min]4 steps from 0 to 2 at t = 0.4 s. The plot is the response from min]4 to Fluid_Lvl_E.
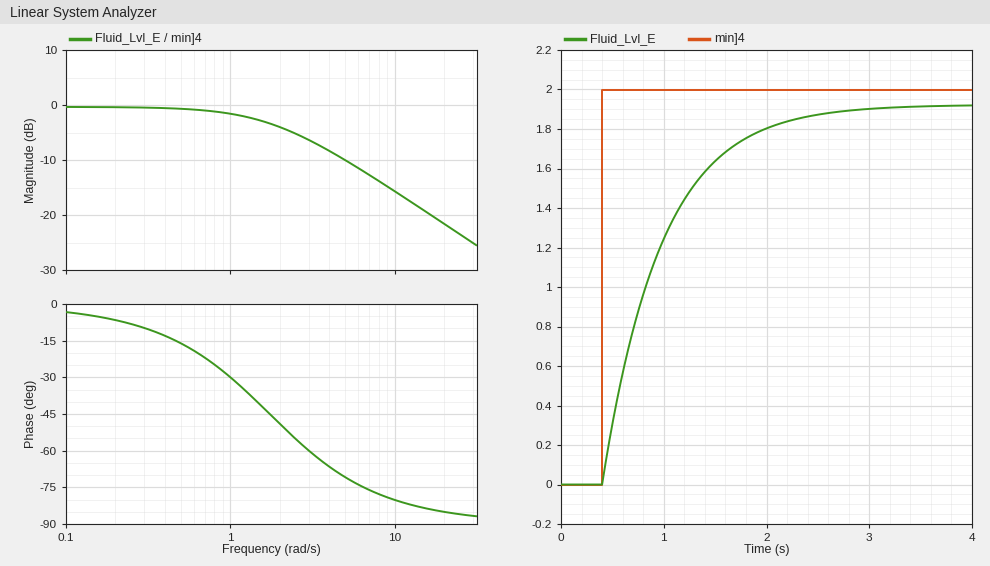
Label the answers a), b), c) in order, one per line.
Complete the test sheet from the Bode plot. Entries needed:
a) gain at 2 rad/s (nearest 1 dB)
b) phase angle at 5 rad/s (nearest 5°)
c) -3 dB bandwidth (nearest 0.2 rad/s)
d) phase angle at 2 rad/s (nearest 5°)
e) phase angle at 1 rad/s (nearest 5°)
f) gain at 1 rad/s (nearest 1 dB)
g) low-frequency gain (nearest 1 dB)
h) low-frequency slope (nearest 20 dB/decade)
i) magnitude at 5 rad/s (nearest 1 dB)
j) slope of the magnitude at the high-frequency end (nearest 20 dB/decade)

a) -4 dB
b) -70°
c) 1.8 rad/s
d) -50°
e) -30°
f) -2 dB
g) 0 dB
h) 0 dB/decade
i) -10 dB
j) -20 dB/decade
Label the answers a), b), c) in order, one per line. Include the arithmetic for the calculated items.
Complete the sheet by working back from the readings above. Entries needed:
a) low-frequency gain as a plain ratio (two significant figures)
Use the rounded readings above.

a) 10^(0 / 20) = 1.0
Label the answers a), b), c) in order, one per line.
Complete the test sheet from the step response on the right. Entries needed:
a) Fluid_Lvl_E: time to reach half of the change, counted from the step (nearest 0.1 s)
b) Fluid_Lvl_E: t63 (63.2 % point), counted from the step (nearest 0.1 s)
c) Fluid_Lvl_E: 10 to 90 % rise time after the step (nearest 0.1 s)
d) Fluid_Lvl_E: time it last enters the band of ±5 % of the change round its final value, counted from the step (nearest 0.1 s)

a) 0.4 s
b) 0.6 s
c) 1.3 s
d) 1.7 s
